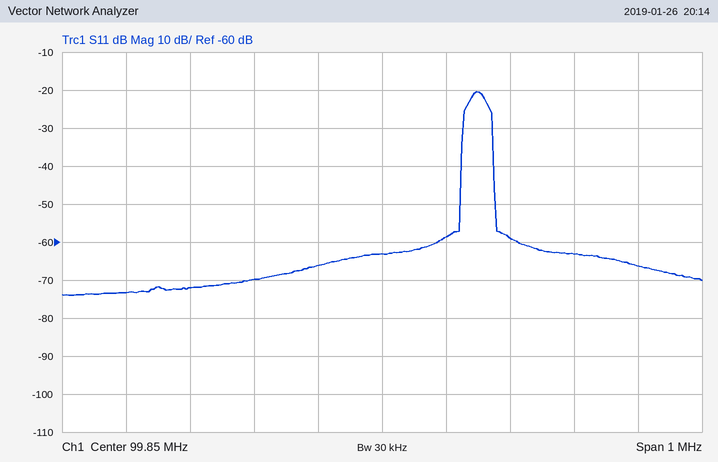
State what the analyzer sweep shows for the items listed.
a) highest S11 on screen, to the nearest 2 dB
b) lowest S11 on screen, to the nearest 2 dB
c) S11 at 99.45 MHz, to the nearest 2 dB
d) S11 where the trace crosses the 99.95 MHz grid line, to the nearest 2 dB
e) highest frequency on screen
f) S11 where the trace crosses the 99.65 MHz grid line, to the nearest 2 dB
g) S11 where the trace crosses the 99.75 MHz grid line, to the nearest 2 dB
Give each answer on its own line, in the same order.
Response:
-20 dB
-74 dB
-74 dB
-58 dB
100.35 MHz
-70 dB
-66 dB
